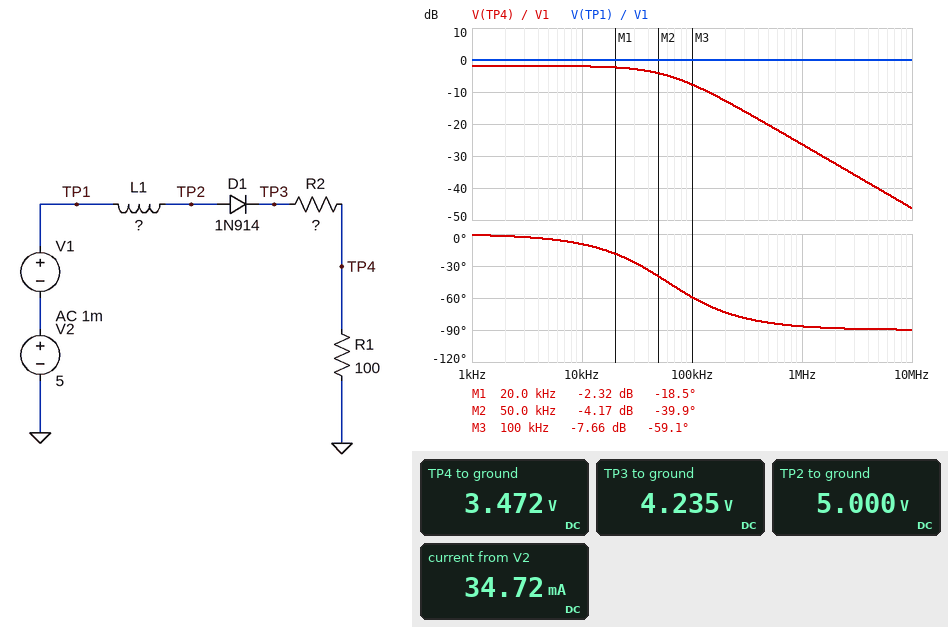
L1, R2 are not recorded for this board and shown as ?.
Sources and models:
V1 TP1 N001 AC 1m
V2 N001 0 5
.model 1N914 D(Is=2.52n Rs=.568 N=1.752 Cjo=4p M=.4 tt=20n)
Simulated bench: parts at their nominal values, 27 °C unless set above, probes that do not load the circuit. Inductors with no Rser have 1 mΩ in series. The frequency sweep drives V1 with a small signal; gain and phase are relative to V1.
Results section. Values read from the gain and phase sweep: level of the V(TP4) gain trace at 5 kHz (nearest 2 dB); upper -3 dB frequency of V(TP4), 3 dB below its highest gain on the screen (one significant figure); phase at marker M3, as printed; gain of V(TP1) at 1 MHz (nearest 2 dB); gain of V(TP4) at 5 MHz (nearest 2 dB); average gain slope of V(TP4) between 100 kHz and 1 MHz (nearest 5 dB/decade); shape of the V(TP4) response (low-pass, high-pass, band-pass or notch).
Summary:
-2 dB
60 kHz
-59.1 deg
0 dB
-40 dB
-20 dB/decade
low-pass
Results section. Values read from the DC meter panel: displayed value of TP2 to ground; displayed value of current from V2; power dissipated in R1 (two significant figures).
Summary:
5.000 V
34.72 mA
120 mW
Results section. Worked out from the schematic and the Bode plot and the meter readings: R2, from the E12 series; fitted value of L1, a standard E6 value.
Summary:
22 Ω
330 µH
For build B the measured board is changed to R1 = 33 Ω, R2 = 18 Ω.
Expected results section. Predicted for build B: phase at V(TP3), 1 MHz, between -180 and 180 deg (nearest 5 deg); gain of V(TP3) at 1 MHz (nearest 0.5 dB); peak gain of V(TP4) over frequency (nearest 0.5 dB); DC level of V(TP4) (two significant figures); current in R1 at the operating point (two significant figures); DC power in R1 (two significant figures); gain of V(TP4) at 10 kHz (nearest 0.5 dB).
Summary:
-90 deg
-32.0 dB
-4.0 dB
2.7 V
82 mA
220 mW
-4.5 dB
